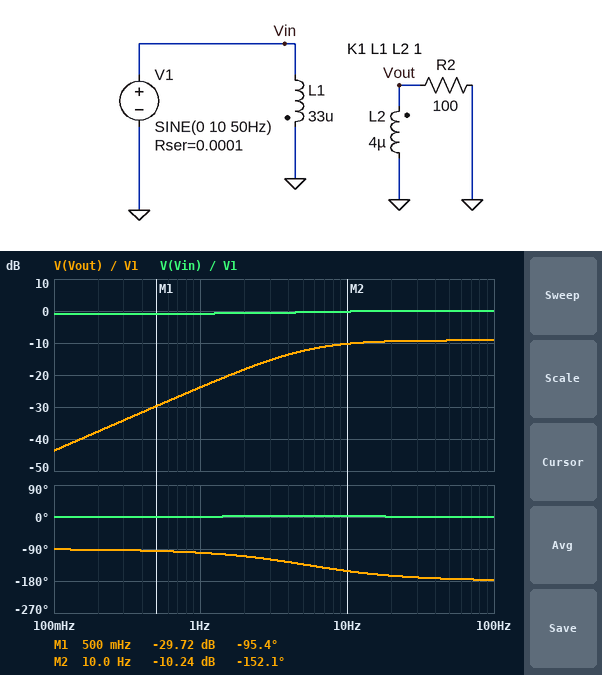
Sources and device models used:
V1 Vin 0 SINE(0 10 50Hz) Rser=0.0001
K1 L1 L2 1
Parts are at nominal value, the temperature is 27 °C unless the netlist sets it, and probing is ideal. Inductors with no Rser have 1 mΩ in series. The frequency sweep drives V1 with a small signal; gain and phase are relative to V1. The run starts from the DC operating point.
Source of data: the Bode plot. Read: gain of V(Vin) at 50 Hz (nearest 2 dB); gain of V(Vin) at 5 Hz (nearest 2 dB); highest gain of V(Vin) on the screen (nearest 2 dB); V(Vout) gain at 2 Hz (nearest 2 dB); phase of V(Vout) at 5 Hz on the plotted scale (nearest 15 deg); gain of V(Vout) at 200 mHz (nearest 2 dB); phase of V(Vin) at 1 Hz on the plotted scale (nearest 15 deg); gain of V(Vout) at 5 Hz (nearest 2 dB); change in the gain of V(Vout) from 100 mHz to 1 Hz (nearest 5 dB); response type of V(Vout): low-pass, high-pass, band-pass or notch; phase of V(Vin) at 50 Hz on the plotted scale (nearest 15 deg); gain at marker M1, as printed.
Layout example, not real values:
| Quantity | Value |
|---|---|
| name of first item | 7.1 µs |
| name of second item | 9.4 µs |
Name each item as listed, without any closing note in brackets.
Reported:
| Quantity | Value |
|---|---|
| gain of V(Vin) at 50 Hz | 0 dB |
| gain of V(Vin) at 5 Hz | 0 dB |
| highest gain of V(Vin) on the screen | 0 dB |
| V(Vout) gain at 2 Hz | -18 dB |
| phase of V(Vout) at 5 Hz on the plotted scale | -135 deg |
| gain of V(Vout) at 200 mHz | -38 dB |
| phase of V(Vin) at 1 Hz on the plotted scale | 0 deg |
| gain of V(Vout) at 5 Hz | -12 dB |
| change in the gain of V(Vout) from 100 mHz to 1 Hz | 20 dB |
| response type of V(Vout): low-pass, high-pass, band-pass or notch | high-pass |
| phase of V(Vin) at 50 Hz on the plotted scale | 0 deg |
| gain at marker M1, as printed | -29.72 dB |
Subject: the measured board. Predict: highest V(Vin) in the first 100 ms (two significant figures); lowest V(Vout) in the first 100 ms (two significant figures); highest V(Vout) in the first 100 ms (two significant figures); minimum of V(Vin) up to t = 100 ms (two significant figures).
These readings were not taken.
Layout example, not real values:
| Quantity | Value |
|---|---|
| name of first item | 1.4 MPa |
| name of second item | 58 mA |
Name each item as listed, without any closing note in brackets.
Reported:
| Quantity | Value |
|---|---|
| highest V(Vin) in the first 100 ms | 10 V |
| lowest V(Vout) in the first 100 ms | -3.4 V |
| highest V(Vout) in the first 100 ms | 3.7 V |
| minimum of V(Vin) up to t = 100 ms | -10 V |
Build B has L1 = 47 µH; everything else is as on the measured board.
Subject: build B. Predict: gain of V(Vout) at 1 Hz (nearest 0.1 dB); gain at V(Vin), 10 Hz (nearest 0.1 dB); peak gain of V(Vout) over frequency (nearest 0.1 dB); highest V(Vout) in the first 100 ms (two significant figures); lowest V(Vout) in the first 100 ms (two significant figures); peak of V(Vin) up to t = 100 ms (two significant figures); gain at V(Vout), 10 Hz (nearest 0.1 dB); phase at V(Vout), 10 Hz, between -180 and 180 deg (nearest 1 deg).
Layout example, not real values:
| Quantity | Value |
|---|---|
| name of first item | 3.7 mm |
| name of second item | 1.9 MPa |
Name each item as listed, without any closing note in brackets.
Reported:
| Quantity | Value |
|---|---|
| gain of V(Vout) at 1 Hz | -22.4 dB |
| gain at V(Vin), 10 Hz | -0.1 dB |
| peak gain of V(Vout) over frequency | -10.7 dB |
| highest V(Vout) in the first 100 ms | 3.1 V |
| lowest V(Vout) in the first 100 ms | -2.9 V |
| peak of V(Vin) up to t = 100 ms | 10 V |
| gain at V(Vout), 10 Hz | -11.3 dB |
| phase at V(Vout), 10 Hz, between -180 and 180 deg | -160 deg |
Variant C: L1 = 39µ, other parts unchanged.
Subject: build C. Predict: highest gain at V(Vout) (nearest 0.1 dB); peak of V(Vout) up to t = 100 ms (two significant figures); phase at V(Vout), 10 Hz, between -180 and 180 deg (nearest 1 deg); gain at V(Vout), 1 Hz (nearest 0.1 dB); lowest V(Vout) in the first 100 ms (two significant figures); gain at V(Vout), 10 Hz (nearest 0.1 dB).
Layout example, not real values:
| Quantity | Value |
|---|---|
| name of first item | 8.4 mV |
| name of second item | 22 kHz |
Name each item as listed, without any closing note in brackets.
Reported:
| Quantity | Value |
|---|---|
| highest gain at V(Vout) | -9.9 dB |
| peak of V(Vout) up to t = 100 ms | 3.4 V |
| phase at V(Vout), 10 Hz, between -180 and 180 deg | -156 deg |
| gain at V(Vout), 1 Hz | -23.1 dB |
| lowest V(Vout) in the first 100 ms | -3.2 V |
| gain at V(Vout), 10 Hz | -10.7 dB |
